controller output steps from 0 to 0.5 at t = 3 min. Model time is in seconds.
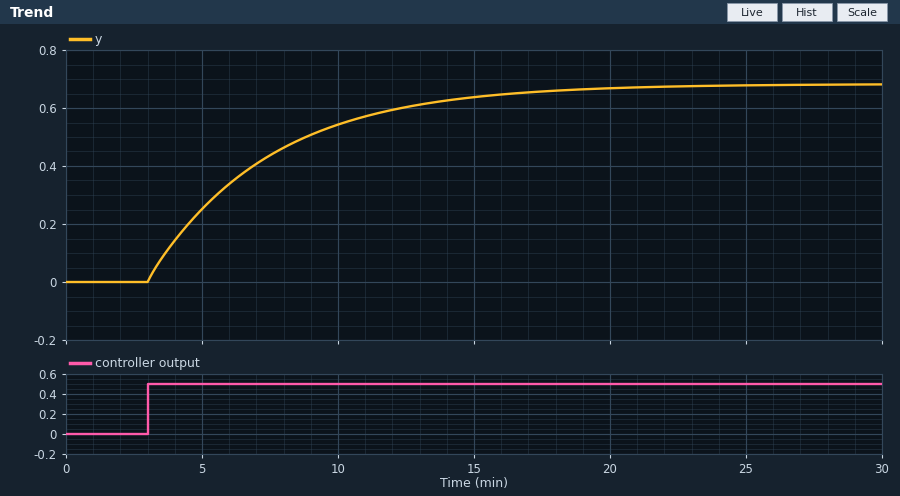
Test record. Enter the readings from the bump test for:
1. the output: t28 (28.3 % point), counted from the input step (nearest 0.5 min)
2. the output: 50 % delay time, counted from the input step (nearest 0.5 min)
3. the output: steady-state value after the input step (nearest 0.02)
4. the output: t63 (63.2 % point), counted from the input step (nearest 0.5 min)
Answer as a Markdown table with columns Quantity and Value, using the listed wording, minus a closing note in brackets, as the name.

| Quantity | Value |
|---|---|
| the output: t28 (28.3 % point), counted from the input step | 1.5 min |
| the output: 50 % delay time, counted from the input step | 3.0 min |
| the output: steady-state value after the input step | 0.68 |
| the output: t63 (63.2 % point), counted from the input step | 4.5 min |
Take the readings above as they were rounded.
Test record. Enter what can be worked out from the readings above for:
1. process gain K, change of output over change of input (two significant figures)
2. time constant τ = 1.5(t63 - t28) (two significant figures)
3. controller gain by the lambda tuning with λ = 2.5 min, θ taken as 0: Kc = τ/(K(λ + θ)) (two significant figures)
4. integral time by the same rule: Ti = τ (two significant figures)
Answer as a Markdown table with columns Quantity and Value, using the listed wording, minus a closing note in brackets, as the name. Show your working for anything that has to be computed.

| Quantity | Value |
|---|---|
| process gain K, change of output over change of input | (0.68 - 0) / 0.5 = 1.4 |
| time constant τ = 1.5(t63 - t28) | 1.5 × (4.5 - 1.5) = 4.5 min |
| controller gain by the lambda tuning with λ = 2.5 min, θ taken as 0: Kc = τ/(K(λ + θ)) | 4.5 / (1.4 × (2.5 + 0)) = 1.3 |
| integral time by the same rule: Ti = τ | 4.5 min |
